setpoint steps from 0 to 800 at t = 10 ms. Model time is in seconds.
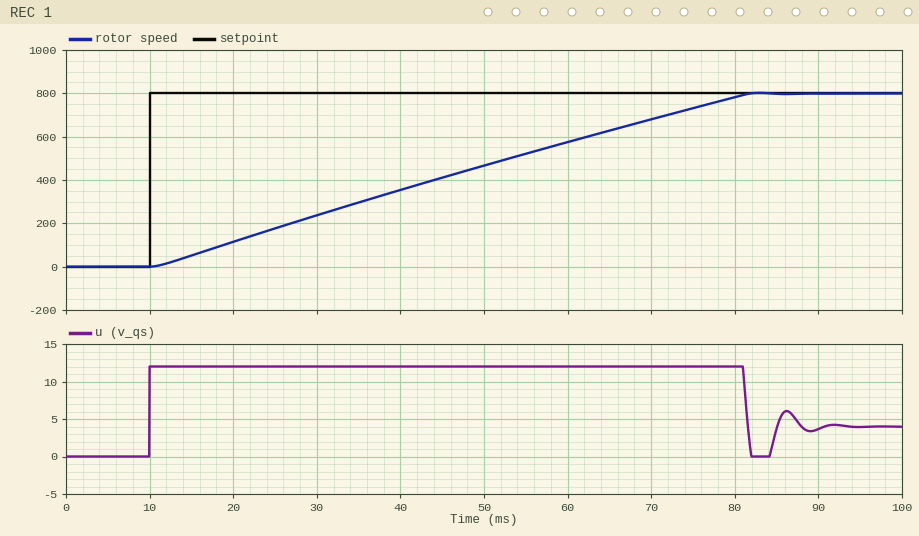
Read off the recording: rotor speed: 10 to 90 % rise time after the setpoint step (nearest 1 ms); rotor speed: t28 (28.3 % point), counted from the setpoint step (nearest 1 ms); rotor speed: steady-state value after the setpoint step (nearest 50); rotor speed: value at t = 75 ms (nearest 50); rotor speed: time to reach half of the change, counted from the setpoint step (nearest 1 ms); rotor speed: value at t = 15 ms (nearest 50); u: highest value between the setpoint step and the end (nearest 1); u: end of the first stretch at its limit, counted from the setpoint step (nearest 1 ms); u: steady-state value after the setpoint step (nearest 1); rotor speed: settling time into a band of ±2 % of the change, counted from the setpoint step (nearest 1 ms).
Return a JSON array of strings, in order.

["57 ms", "19 ms", "800", "750", "34 ms", "50", "12", "71 ms", "4", "70 ms"]
